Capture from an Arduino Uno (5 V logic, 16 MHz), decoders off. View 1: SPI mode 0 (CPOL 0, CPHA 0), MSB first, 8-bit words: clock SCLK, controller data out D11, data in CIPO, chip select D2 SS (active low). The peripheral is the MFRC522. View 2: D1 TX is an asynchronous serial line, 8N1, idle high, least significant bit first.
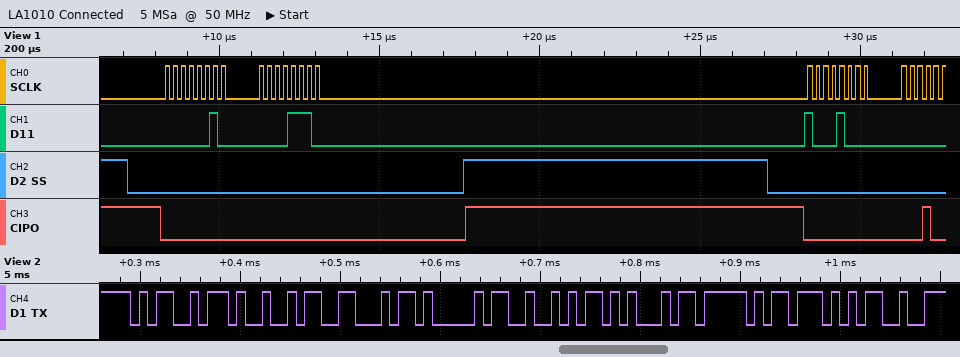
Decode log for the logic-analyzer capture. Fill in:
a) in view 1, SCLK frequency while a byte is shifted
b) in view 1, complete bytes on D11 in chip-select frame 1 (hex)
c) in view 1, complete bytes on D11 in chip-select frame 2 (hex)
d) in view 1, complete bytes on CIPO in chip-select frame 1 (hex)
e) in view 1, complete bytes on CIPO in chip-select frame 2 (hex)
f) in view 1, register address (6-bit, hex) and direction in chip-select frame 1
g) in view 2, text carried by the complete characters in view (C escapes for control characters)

4 MHz
02 0E
88
00 00
00
0x01 write
"MIFARE_W"
